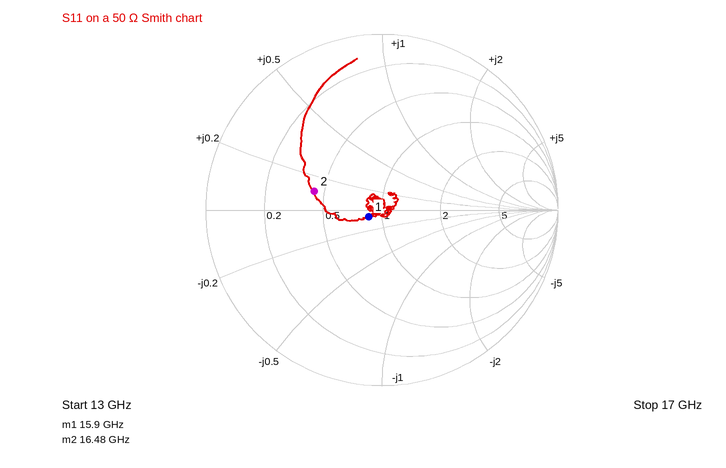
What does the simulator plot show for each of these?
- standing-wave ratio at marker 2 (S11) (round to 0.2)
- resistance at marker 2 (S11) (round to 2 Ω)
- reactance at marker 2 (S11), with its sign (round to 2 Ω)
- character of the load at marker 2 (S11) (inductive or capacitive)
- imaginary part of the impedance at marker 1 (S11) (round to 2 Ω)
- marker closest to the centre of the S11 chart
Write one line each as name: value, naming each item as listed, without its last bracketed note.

standing-wave ratio at marker 2 (S11): 2.4
resistance at marker 2 (S11): 22 Ω
reactance at marker 2 (S11), with its sign: +6 Ω
character of the load at marker 2 (S11): inductive
imaginary part of the impedance at marker 1 (S11): -4 Ω
marker closest to the centre of the S11 chart: marker 1
